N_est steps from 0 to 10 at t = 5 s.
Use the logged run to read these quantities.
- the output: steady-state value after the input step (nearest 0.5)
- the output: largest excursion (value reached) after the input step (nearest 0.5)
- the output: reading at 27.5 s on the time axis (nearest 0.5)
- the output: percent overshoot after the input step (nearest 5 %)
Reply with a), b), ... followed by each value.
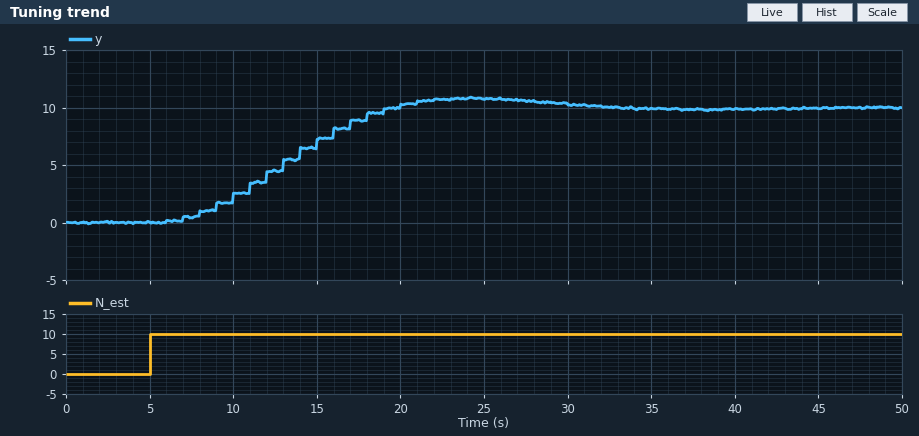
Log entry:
a) 10.0
b) 11.0
c) 10.5
d) 10 %
